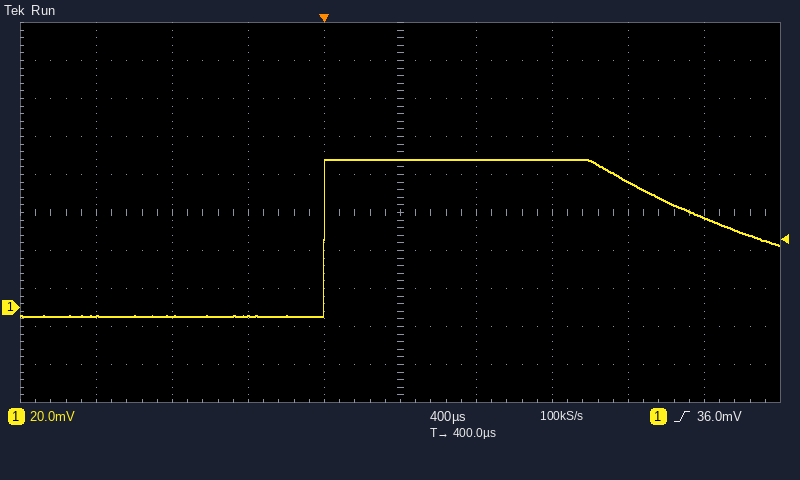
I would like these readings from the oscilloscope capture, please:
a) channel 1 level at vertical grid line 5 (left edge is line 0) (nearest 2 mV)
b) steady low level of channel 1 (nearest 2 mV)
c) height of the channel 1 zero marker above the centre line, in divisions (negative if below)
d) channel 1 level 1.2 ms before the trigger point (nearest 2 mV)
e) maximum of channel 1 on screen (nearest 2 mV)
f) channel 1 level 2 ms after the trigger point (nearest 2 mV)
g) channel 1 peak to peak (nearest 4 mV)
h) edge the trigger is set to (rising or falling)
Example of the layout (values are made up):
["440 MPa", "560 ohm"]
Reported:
["78 mV", "-4 mV", "-2.5 div", "-4 mV", "78 mV", "48 mV", "84 mV", "rising"]
